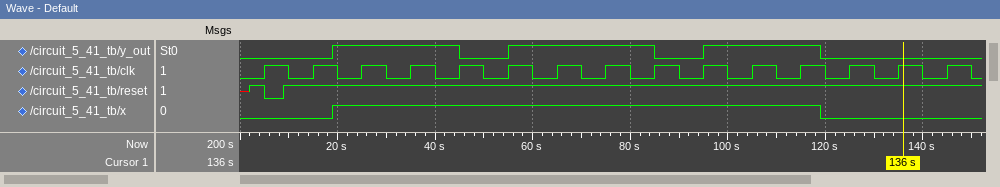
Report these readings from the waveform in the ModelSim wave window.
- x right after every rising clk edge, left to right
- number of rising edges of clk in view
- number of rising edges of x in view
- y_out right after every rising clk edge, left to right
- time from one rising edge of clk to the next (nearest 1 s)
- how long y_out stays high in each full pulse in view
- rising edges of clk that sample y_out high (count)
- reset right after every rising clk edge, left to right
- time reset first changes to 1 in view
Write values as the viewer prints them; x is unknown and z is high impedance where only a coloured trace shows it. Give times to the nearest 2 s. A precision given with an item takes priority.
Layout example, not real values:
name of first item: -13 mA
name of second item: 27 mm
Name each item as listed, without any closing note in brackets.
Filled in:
x right after every rising clk edge, left to right: 0 0 1 1 1 1 1 1 1 1 1 1 0 0 0
number of rising edges of clk in view: 15
number of rising edges of x in view: 1
y_out right after every rising clk edge, left to right: 0 0 1 1 0 1 1 1 0 1 1 1 0 0 0
time from one rising edge of clk to the next: 10 s
how long y_out stays high in each full pulse in view: 26 s, 30 s, 24 s
rising edges of clk that sample y_out high: 8
reset right after every rising clk edge, left to right: 0 1 1 1 1 1 1 1 1 1 1 1 1 1 1
time reset first changes to 1 in view: 2 s
